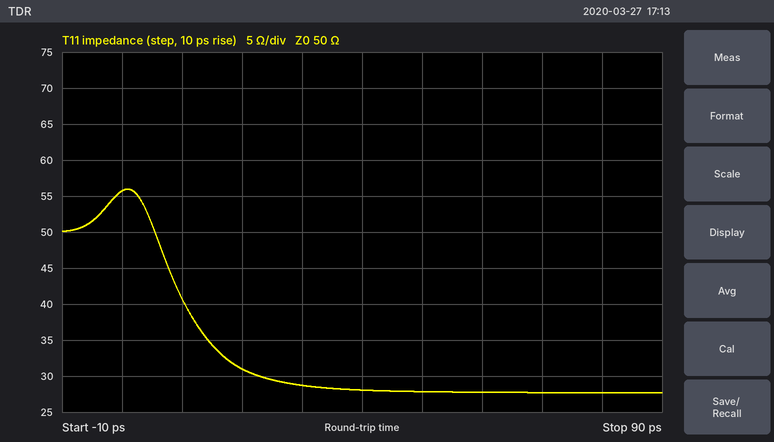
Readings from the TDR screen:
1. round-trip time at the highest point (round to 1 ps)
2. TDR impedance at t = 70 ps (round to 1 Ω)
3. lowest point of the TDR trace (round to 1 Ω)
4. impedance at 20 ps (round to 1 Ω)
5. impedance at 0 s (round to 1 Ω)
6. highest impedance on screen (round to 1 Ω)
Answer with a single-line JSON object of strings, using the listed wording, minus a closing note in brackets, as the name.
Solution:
{"round-trip time at the highest point": "1 ps", "TDR impedance at t = 70 ps": "28 Ω", "lowest point of the TDR trace": "28 Ω", "impedance at 20 ps": "31 Ω", "impedance at 0 s": "56 Ω", "highest impedance on screen": "56 Ω"}
